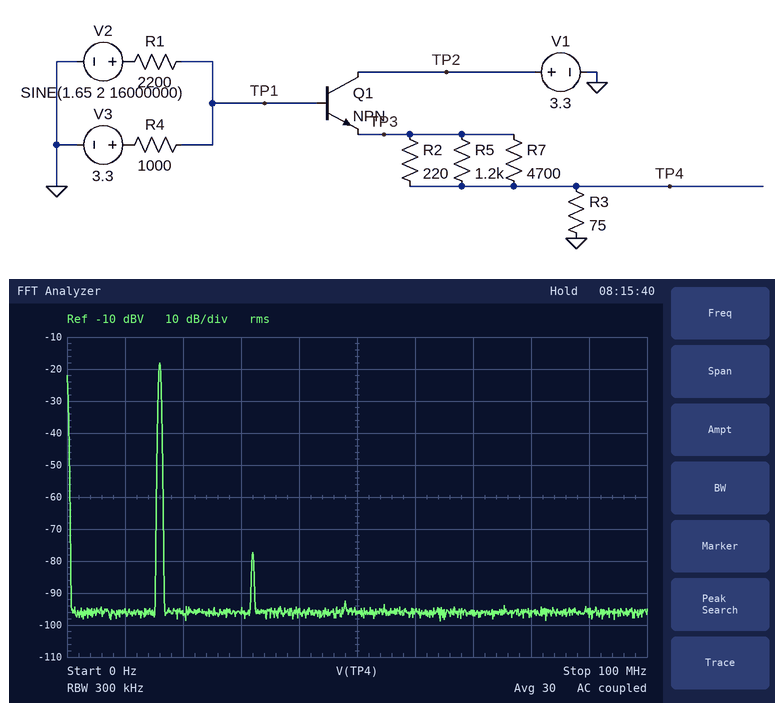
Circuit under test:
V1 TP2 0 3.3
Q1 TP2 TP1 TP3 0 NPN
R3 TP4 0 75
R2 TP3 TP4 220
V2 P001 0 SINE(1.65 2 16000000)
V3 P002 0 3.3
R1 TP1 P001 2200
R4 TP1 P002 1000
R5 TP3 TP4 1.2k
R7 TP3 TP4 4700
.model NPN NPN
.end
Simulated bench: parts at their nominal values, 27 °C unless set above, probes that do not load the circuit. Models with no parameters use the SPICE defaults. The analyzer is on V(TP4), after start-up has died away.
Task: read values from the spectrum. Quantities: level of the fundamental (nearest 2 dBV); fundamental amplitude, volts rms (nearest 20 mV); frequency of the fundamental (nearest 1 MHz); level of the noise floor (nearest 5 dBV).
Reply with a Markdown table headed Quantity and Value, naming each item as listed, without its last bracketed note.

| Quantity | Value |
|---|---|
| level of the fundamental | -18 dBV |
| fundamental amplitude, volts rms | 120 mV |
| frequency of the fundamental | 16 MHz |
| level of the noise floor | -95 dBV |
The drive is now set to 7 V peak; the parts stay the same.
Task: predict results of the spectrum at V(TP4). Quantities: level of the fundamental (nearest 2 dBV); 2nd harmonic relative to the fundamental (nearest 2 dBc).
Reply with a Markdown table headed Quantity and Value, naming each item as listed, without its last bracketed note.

| Quantity | Value |
|---|---|
| level of the fundamental | -8 dBV |
| 2nd harmonic relative to the fundamental | -20 dBc |
